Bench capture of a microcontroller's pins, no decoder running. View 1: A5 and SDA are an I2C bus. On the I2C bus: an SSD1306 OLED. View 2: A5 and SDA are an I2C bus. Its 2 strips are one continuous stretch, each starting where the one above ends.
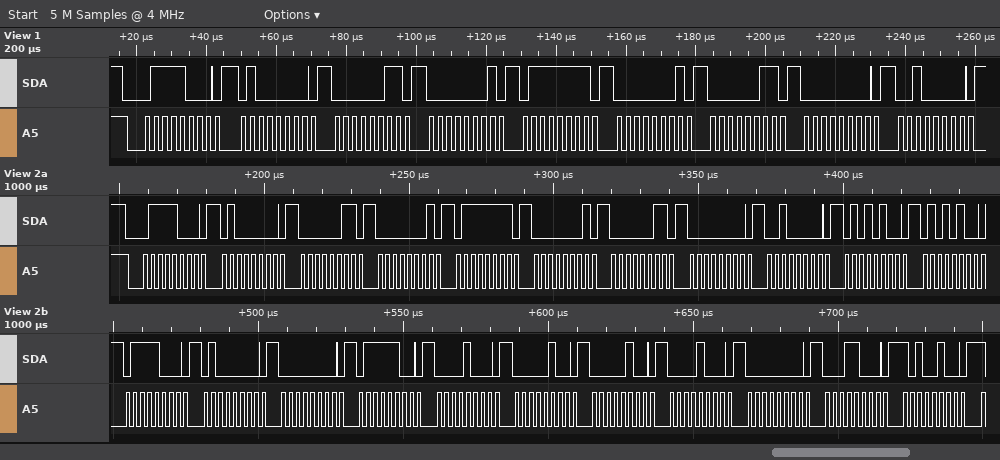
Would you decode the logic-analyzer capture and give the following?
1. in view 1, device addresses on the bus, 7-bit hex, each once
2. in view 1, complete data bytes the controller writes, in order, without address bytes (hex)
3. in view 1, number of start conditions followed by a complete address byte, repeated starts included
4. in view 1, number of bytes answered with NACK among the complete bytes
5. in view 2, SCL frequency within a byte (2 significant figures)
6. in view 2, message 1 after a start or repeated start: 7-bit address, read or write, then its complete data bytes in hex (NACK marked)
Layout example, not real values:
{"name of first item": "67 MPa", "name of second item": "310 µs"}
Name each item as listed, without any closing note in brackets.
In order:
{"in view 1, device addresses on the bus, 7-bit hex, each once": "0x3C", "in view 1, complete data bytes the controller writes, in order, without address bytes": "40 03 01 7F 01 03 00 20", "in view 1, number of start conditions followed by a complete address byte, repeated starts included": "1", "in view 1, number of bytes answered with NACK among the complete bytes": "0", "in view 2, SCL frequency within a byte": "400 kHz", "in view 2, message 1 after a start or repeated start: 7-bit address, read or write, then its complete data bytes in hex": "0x3C write: 40 03 01 7F 01 03 00 20 54 54 78 40 00 7C 08 04 04 08 00 18 A4"}
